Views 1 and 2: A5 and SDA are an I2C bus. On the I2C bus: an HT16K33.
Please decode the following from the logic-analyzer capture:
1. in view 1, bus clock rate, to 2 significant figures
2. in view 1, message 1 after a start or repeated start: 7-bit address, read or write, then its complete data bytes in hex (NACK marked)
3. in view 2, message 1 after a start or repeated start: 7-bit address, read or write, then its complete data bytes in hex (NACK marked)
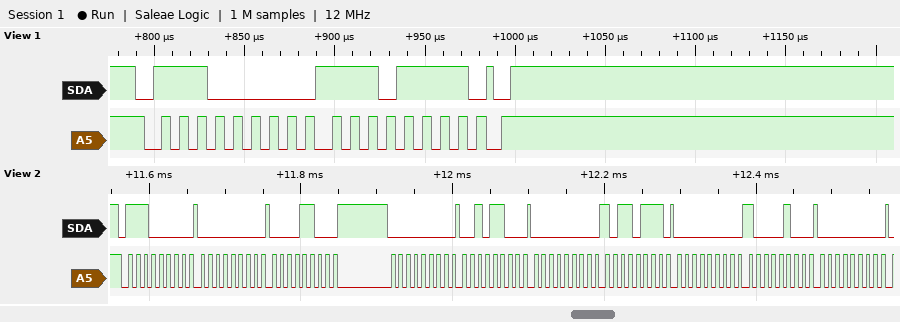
100 kHz
0x70 write: EF
0x70 write: 00 0C 00 2C 00 B7 00 84 00
